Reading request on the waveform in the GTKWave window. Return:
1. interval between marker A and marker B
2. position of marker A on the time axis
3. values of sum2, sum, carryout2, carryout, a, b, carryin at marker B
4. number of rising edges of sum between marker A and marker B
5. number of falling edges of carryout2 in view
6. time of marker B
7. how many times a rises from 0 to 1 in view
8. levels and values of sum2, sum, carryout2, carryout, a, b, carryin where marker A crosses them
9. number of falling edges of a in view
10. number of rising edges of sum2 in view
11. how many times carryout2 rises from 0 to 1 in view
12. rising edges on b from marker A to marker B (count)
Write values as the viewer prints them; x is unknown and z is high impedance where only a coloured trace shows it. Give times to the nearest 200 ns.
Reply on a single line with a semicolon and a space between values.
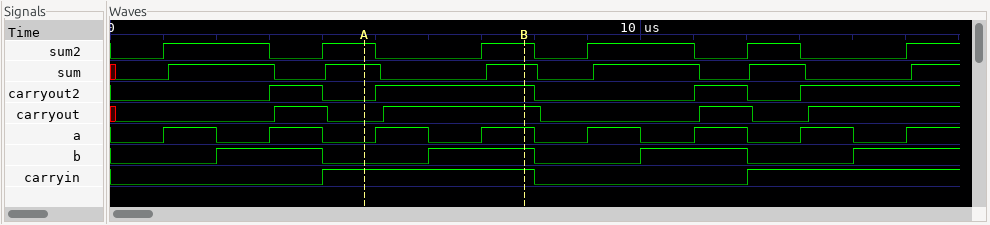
3000 ns; 4800 ns; sum2=1, sum=1, carryout2=1, carryout=1, a=1, b=1, carryin=1; 1; 3; 7800 ns; 8; sum2=1, sum=1, carryout2=0, carryout=0, a=0, b=0, carryin=1; 7; 6; 4; 1
